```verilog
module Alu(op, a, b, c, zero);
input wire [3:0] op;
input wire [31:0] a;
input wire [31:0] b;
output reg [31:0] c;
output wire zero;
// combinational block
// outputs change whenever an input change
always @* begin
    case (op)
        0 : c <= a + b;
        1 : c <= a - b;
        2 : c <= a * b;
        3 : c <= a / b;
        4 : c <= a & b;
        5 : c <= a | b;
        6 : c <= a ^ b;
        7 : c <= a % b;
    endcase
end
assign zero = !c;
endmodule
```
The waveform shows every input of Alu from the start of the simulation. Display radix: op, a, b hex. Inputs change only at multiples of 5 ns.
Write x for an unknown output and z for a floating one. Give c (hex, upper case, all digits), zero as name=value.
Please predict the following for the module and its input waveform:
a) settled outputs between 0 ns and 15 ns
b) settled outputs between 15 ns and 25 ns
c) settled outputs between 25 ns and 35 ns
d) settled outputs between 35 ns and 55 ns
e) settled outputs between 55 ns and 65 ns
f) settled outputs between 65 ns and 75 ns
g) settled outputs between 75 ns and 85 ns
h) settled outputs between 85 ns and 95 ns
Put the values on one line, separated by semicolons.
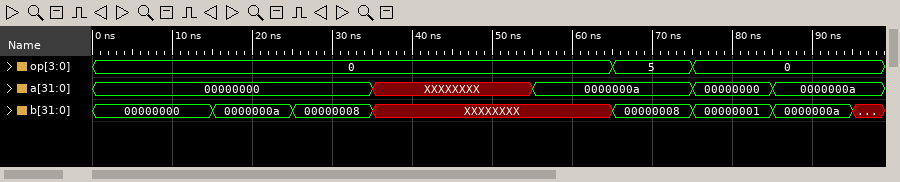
c=00000000, zero=1; c=0000000A, zero=0; c=00000008, zero=0; c=x, zero=x; c=x, zero=x; c=0000000A, zero=0; c=00000001, zero=0; c=00000014, zero=0
